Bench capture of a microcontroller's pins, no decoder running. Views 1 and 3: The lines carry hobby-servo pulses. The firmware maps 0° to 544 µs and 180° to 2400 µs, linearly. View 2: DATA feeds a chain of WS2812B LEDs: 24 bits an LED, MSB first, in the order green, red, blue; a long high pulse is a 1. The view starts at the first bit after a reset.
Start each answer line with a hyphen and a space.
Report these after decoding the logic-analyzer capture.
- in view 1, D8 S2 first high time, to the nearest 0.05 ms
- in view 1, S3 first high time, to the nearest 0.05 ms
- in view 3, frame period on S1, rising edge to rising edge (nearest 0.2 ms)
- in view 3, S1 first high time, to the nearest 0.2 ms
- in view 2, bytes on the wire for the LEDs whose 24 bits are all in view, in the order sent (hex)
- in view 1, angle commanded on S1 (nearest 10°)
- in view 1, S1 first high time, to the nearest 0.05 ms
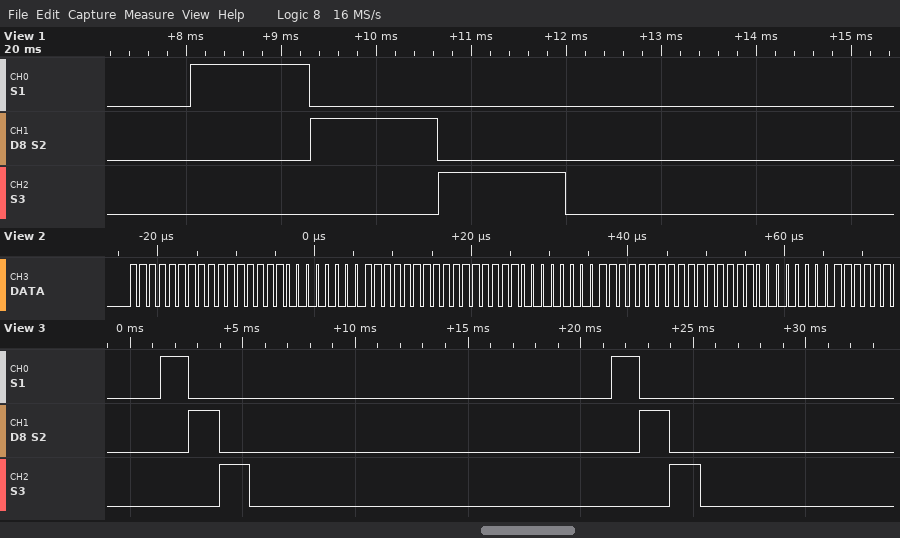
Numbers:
- 1.35 ms
- 1.35 ms
- 20.0 ms
- 1.2 ms
- FF FF 00 FF FF 00 FF FF 00
- 70°
- 1.25 ms
